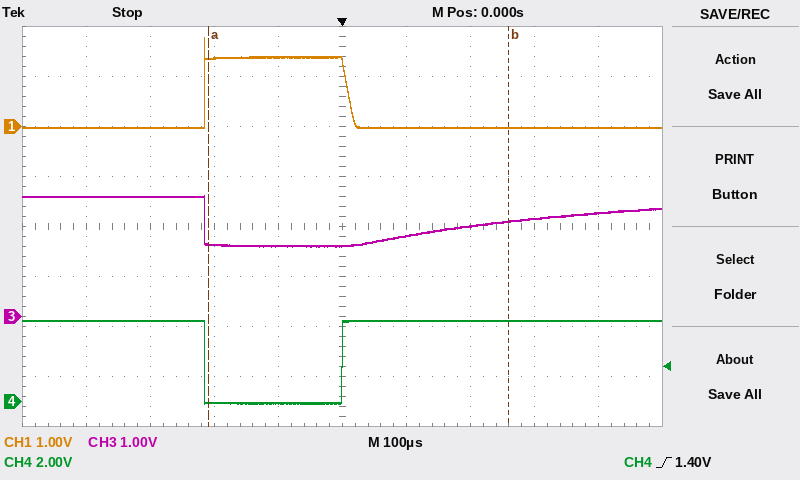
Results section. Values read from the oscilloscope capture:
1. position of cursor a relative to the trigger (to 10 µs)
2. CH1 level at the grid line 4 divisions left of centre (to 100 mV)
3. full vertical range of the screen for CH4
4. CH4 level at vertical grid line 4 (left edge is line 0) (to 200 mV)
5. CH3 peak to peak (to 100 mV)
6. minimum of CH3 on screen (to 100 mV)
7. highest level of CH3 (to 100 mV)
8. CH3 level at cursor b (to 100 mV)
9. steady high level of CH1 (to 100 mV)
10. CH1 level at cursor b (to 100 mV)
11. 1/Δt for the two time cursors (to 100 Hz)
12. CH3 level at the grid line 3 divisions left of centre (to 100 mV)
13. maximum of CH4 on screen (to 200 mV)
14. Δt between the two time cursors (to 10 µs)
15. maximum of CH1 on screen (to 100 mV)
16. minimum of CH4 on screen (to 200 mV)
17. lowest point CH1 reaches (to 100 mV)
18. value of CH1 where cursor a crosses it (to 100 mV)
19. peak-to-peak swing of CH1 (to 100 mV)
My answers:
-210 µs
0.0 V
16 V
0.0 V
1.0 V
1.4 V
2.4 V
1.9 V
1.4 V
0.0 V
2.1 kHz
2.4 V
3.2 V
470 µs
1.8 V
0.0 V
0.0 V
1.4 V
1.8 V
